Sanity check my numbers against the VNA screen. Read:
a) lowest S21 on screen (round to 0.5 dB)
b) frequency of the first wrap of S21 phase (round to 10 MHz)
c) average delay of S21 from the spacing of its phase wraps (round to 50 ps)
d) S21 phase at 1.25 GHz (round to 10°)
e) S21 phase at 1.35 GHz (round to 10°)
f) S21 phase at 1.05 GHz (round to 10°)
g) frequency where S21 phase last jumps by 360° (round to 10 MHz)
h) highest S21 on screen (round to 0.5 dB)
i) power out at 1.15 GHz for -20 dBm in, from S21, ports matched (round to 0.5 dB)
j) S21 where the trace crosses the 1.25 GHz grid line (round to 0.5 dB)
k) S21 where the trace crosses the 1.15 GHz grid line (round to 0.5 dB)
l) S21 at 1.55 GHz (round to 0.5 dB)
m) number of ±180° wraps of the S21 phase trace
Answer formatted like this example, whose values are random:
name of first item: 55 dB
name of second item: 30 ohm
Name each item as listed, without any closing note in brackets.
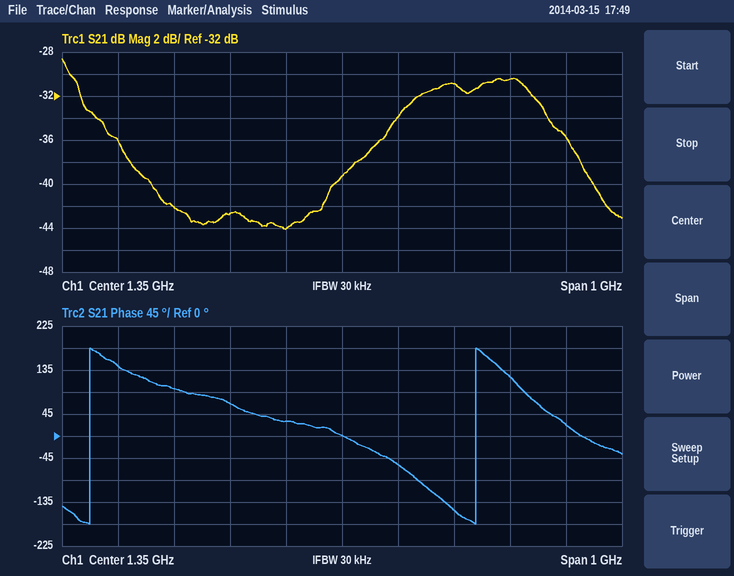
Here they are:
lowest S21 on screen: -44.0 dB
frequency of the first wrap of S21 phase: 900 MHz
average delay of S21 from the spacing of its phase wraps: 1.45 ns
S21 phase at 1.25 GHz: 30°
S21 phase at 1.35 GHz: 0°
S21 phase at 1.05 GHz: 100°
frequency where S21 phase last jumps by 360°: 1.59 GHz
highest S21 on screen: -28.5 dB
power out at 1.15 GHz for -20 dBm in, from S21, ports matched: -62.5 dBm
S21 where the trace crosses the 1.25 GHz grid line: -44.0 dB
S21 where the trace crosses the 1.15 GHz grid line: -42.5 dB
S21 at 1.55 GHz: -31.0 dB
number of ±180° wraps of the S21 phase trace: 2
